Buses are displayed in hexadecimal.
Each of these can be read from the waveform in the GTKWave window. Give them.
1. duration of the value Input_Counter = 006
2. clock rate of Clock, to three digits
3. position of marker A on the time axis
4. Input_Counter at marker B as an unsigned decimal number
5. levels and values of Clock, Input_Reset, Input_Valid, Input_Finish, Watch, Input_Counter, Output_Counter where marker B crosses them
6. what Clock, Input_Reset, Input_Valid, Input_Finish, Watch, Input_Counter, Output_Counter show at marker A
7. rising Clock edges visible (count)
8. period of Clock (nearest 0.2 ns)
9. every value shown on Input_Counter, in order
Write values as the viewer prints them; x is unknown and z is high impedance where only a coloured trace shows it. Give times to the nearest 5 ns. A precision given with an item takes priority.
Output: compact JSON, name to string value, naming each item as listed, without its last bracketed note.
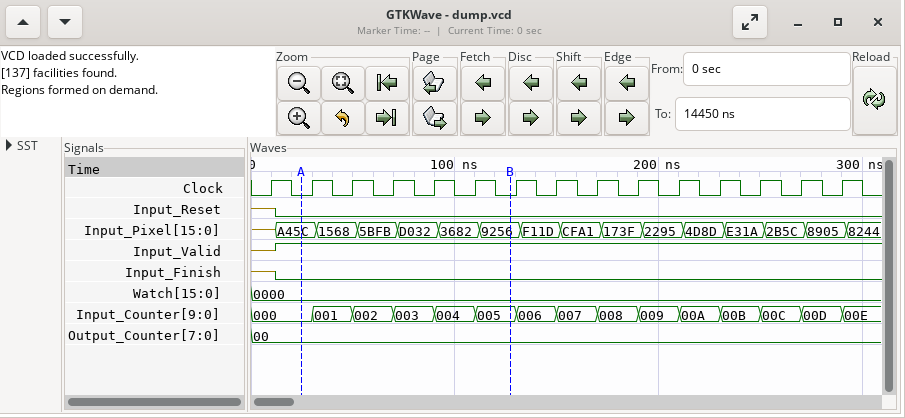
{"duration of the value Input_Counter = 006": "20 ns", "clock rate of Clock, to three digits": "50.0 MHz", "position of marker A on the time axis": "25 ns", "Input_Counter at marker B as an unsigned decimal number": "5", "levels and values of Clock, Input_Reset, Input_Valid, Input_Finish, Watch, Input_Counter, Output_Counter where marker B crosses them": "Clock=0, Input_Reset=0, Input_Valid=1, Input_Finish=0, Watch=0000, Input_Counter=005, Output_Counter=00", "what Clock, Input_Reset, Input_Valid, Input_Finish, Watch, Input_Counter, Output_Counter show at marker A": "Clock=0, Input_Reset=0, Input_Valid=1, Input_Finish=0, Watch=0000, Input_Counter=000, Output_Counter=00", "rising Clock edges visible": "15", "period of Clock": "20 ns", "every value shown on Input_Counter, in order": "000, 001, 002, 003, 004, 005, 006, 007, 008, 009, 00A, 00B, 00C, 00D, 00E"}
